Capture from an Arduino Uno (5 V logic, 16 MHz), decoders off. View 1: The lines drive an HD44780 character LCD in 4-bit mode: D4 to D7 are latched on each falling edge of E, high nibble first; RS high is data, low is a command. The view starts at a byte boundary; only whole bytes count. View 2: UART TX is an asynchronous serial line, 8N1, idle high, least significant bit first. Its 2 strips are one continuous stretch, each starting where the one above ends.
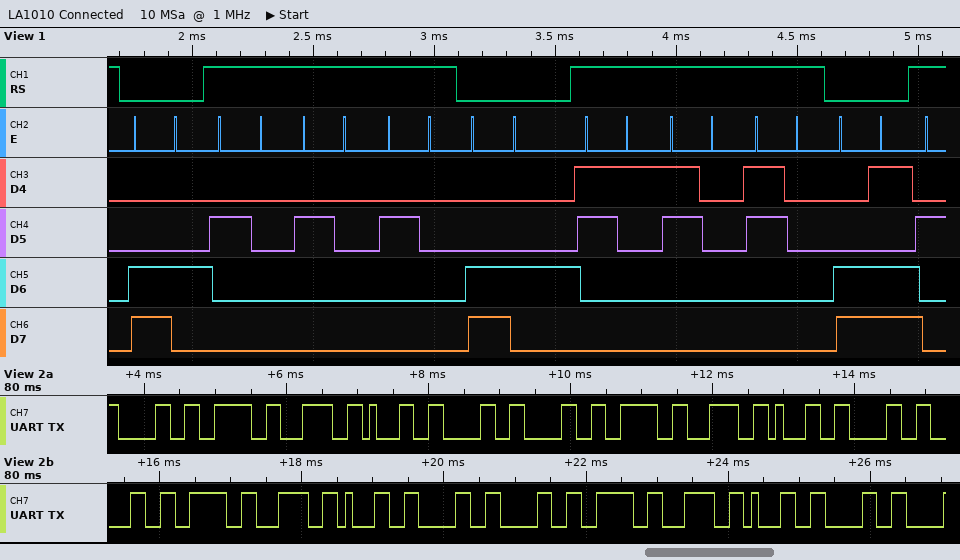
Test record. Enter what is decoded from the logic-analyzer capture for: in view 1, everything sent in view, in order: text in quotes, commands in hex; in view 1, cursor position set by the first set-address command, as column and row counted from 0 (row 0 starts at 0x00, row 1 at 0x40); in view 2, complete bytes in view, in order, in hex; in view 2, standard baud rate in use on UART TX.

0xC4 "   " 0xC4 "100" 0xCD
column 4, row 1
30 3E 3C 31 30 30 3E 3C 31 30 30 3E 3C 31 30 30 3E 3C 31 30
9600 baud
